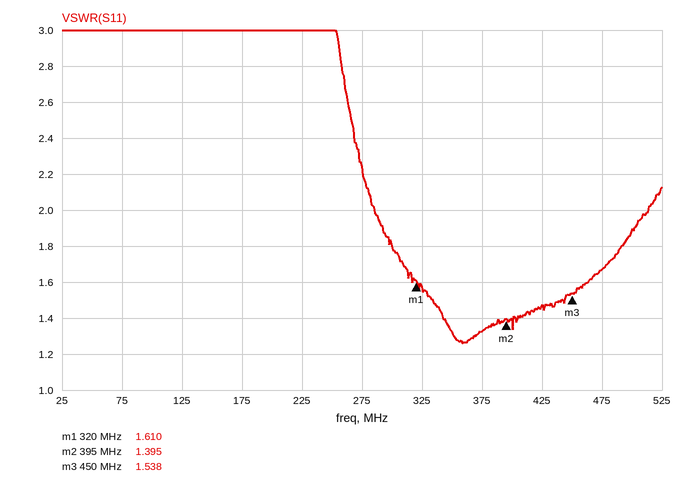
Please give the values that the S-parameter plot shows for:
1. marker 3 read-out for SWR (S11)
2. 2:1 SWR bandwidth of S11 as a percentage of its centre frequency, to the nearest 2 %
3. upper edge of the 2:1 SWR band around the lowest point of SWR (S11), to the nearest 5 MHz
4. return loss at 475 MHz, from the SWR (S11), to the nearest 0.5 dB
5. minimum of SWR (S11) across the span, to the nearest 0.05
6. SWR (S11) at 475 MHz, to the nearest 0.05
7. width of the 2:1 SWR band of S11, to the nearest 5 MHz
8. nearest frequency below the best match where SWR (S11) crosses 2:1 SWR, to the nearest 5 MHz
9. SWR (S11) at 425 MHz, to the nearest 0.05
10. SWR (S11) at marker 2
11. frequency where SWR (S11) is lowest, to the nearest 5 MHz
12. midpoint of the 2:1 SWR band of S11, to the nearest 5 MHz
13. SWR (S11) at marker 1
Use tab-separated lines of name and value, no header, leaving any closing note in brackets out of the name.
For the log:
marker 3 read-out for SWR	1.538
2:1 SWR bandwidth of S11 as a percentage of its centre frequency, to the nearest 2 %	58 %
upper edge of the 2:1 SWR band around the lowest point of SWR (S11), to the nearest 5 MHz	515 MHz
return loss at 475 MHz, from the SWR (S11), to the nearest 0.5 dB	12.0 dB
minimum of SWR (S11) across the span, to the nearest 0.05	1.25
SWR (S11) at 475 MHz, to the nearest 0.05	1.65
width of the 2:1 SWR band of S11, to the nearest 5 MHz	230 MHz
nearest frequency below the best match where SWR (S11) crosses 2:1 SWR, to the nearest 5 MHz	285 MHz
SWR (S11) at 425 MHz, to the nearest 0.05	1.45
SWR (S11) at marker 2	1.395
frequency where SWR (S11) is lowest, to the nearest 5 MHz	360 MHz
midpoint of the 2:1 SWR band of S11, to the nearest 5 MHz	400 MHz
SWR (S11) at marker 1	1.610
